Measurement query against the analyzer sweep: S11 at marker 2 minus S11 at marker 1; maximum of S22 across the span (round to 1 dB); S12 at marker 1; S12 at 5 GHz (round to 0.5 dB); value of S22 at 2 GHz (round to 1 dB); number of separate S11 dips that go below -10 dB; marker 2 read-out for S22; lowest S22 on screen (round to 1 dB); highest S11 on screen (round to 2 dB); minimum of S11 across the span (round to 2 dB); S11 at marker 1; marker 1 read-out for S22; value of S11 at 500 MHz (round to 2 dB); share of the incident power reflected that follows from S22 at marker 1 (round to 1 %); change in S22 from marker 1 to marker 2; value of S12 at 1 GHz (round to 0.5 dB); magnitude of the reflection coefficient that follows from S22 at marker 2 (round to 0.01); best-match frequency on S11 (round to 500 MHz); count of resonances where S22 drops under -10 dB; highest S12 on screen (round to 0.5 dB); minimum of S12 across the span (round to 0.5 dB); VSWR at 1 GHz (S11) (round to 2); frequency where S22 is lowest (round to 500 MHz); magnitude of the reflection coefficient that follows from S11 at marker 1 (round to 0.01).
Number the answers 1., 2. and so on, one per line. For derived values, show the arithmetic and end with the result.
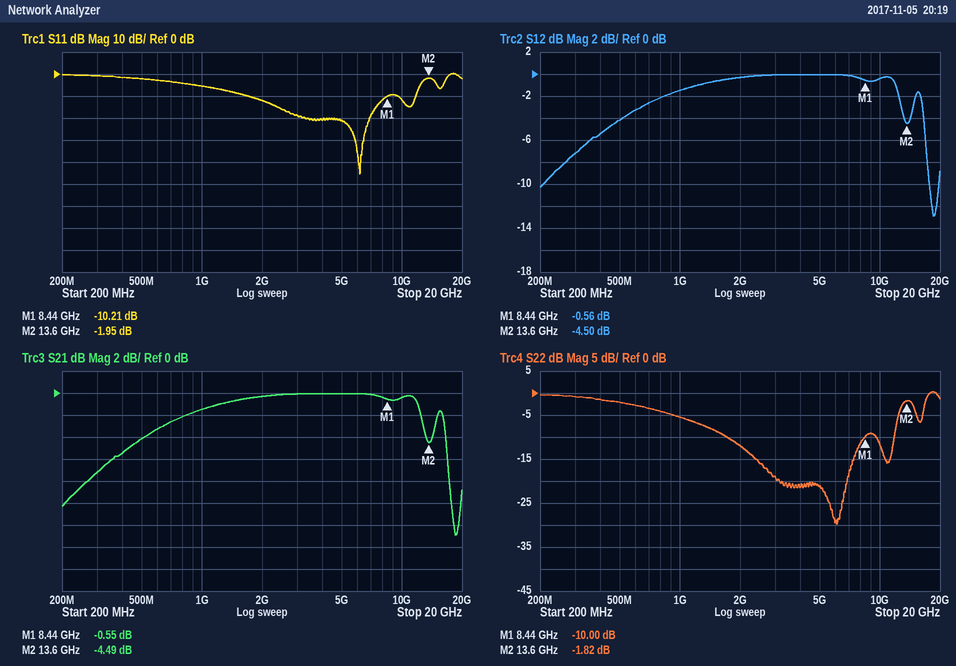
1. -1.95 − (-10.21) = 8.26 dB
2. 0 dB
3. -0.56 dB
4. 0.0 dB
5. -12 dB
6. 2
7. -1.82 dB
8. -30 dB
9. 0 dB
10. -46 dB
11. -10.21 dB
12. -10.00 dB
13. -2 dB
14. 10^(-10/10) ≈ 10 %
15. -1.82 − (-10) = 8.18 dB
16. -1.5 dB
17. 10^(-1.82/20) ≈ 0.81
18. 6.0 GHz
19. 2
20. 0.0 dB
21. -13.0 dB
22. |Γ| = 10^(-6/20) = 0.5012; VSWR = (1 + 0.5012)/(1 − 0.5012) ≈ 3.01, so 4 to the nearest 2
23. 6.0 GHz
24. 10^(-10.21/20) ≈ 0.31
